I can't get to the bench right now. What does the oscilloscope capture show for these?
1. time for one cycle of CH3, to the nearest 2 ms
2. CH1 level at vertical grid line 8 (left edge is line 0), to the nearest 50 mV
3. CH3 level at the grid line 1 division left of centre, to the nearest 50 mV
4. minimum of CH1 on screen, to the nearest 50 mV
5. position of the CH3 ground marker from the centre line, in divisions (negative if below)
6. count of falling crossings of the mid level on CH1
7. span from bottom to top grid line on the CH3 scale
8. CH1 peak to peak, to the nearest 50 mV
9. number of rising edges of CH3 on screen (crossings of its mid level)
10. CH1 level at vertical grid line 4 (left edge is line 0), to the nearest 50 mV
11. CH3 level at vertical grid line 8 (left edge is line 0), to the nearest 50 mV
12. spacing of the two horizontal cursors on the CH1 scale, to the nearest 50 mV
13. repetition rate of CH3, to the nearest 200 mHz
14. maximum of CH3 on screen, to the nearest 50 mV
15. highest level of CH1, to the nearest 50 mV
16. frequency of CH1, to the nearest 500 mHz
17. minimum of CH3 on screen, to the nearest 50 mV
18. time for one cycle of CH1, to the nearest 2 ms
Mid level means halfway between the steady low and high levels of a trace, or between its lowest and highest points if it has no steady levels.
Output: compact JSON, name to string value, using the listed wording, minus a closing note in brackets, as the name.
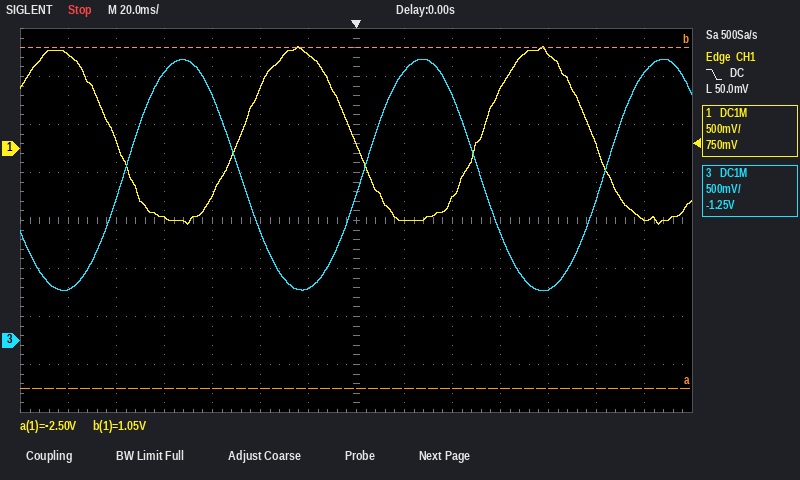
{"time for one cycle of CH3, to the nearest 2 ms": "100 ms", "CH1 level at vertical grid line 8 (left edge is line 0), to the nearest 50 mV": "-750 mV", "CH3 level at the grid line 1 division left of centre, to the nearest 50 mV": "550 mV", "minimum of CH1 on screen, to the nearest 50 mV": "-800 mV", "position of the CH3 ground marker from the centre line, in divisions": "-2.5 div", "count of falling crossings of the mid level on CH1": "3", "span from bottom to top grid line on the CH3 scale": "4 V", "CH1 peak to peak, to the nearest 50 mV": "1.85 V", "number of rising edges of CH3 on screen": "3", "CH1 level at vertical grid line 4 (left edge is line 0), to the nearest 50 mV": "-500 mV", "CH3 level at vertical grid line 8 (left edge is line 0), to the nearest 50 mV": "2.80 V", "spacing of the two horizontal cursors on the CH1 scale, to the nearest 50 mV": "3.55 V", "repetition rate of CH3, to the nearest 200 mHz": "10.0 Hz", "maximum of CH3 on screen, to the nearest 50 mV": "2.95 V", "highest level of CH1, to the nearest 50 mV": "1.05 V", "frequency of CH1, to the nearest 500 mHz": "10.0 Hz", "minimum of CH3 on screen, to the nearest 50 mV": "500 mV", "time for one cycle of CH1, to the nearest 2 ms": "100 ms"}
